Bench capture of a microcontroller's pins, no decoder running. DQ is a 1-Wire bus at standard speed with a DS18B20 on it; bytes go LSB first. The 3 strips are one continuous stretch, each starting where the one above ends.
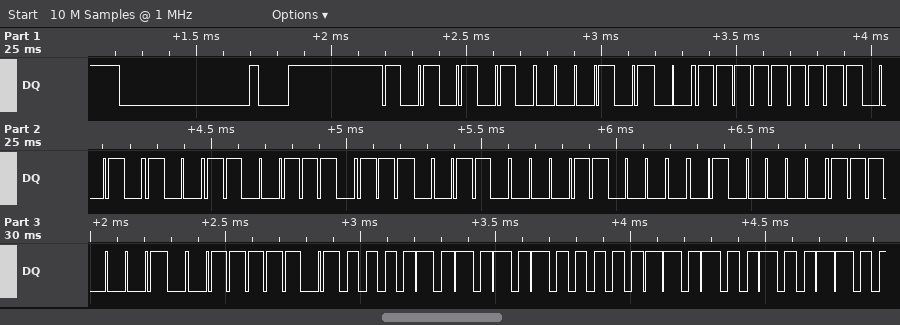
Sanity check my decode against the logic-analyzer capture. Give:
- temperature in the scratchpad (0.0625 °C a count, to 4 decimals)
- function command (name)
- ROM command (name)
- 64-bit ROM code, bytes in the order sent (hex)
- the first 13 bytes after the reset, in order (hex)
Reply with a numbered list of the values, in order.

1. 85.0000 °C
2. Read Scratchpad
3. Match ROM
4. 28 FF 29 73 67 18 04 47
5. 55 28 FF 29 73 67 18 04 47 BE 50 05 4B
